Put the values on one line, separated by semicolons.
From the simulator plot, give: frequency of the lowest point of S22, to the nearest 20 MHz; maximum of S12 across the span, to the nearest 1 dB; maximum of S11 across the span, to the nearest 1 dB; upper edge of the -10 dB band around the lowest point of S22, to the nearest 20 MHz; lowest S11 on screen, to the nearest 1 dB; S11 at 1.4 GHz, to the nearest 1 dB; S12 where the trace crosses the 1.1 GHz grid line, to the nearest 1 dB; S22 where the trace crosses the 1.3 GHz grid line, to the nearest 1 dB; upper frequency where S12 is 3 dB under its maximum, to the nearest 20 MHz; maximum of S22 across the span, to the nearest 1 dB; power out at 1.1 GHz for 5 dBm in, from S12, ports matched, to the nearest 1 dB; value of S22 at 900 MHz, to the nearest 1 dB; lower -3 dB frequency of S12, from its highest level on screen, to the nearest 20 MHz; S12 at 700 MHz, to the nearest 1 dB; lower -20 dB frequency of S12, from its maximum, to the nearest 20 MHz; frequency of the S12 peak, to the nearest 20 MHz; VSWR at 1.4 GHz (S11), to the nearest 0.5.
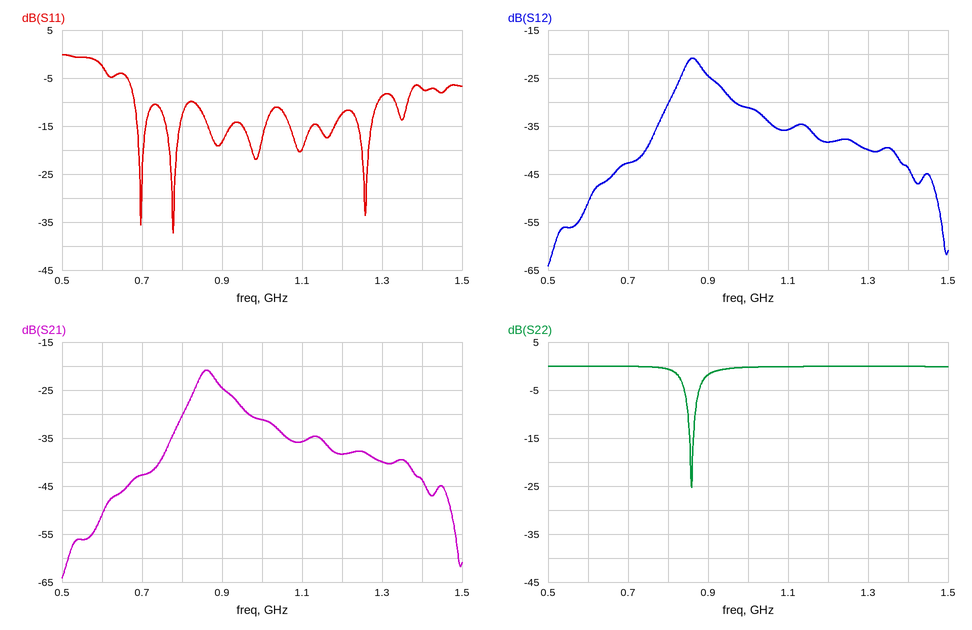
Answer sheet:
860 MHz; -21 dB; 0 dB; 860 MHz; -37 dB; -7 dB; -36 dB; 0 dB; 900 MHz; 0 dB; -31 dBm; -2 dB; 840 MHz; -43 dB; 740 MHz; 860 MHz; 2.5
